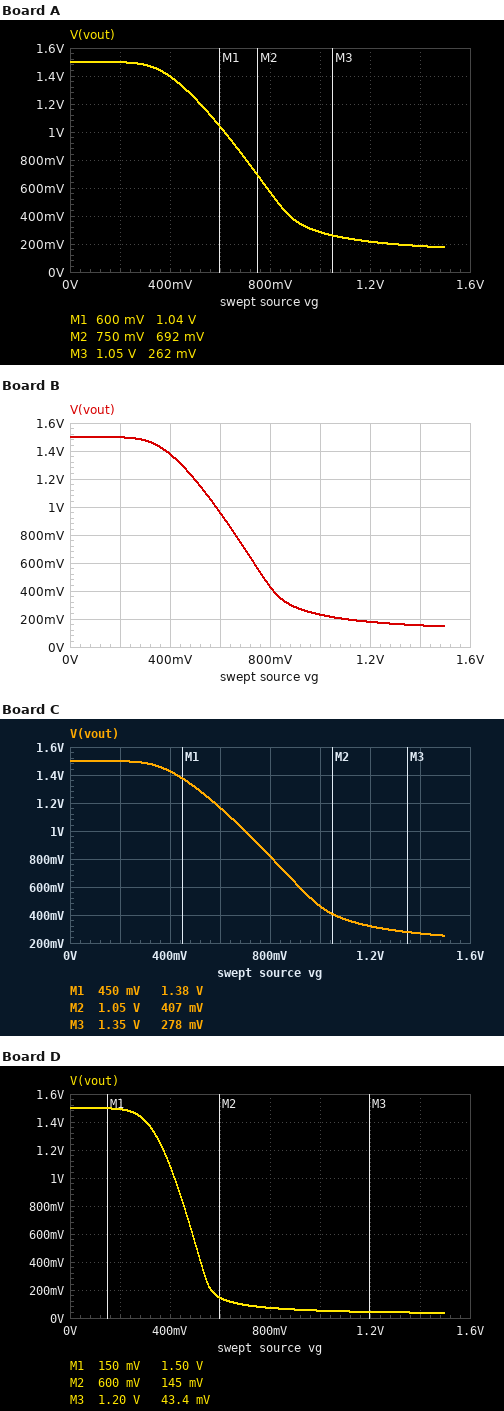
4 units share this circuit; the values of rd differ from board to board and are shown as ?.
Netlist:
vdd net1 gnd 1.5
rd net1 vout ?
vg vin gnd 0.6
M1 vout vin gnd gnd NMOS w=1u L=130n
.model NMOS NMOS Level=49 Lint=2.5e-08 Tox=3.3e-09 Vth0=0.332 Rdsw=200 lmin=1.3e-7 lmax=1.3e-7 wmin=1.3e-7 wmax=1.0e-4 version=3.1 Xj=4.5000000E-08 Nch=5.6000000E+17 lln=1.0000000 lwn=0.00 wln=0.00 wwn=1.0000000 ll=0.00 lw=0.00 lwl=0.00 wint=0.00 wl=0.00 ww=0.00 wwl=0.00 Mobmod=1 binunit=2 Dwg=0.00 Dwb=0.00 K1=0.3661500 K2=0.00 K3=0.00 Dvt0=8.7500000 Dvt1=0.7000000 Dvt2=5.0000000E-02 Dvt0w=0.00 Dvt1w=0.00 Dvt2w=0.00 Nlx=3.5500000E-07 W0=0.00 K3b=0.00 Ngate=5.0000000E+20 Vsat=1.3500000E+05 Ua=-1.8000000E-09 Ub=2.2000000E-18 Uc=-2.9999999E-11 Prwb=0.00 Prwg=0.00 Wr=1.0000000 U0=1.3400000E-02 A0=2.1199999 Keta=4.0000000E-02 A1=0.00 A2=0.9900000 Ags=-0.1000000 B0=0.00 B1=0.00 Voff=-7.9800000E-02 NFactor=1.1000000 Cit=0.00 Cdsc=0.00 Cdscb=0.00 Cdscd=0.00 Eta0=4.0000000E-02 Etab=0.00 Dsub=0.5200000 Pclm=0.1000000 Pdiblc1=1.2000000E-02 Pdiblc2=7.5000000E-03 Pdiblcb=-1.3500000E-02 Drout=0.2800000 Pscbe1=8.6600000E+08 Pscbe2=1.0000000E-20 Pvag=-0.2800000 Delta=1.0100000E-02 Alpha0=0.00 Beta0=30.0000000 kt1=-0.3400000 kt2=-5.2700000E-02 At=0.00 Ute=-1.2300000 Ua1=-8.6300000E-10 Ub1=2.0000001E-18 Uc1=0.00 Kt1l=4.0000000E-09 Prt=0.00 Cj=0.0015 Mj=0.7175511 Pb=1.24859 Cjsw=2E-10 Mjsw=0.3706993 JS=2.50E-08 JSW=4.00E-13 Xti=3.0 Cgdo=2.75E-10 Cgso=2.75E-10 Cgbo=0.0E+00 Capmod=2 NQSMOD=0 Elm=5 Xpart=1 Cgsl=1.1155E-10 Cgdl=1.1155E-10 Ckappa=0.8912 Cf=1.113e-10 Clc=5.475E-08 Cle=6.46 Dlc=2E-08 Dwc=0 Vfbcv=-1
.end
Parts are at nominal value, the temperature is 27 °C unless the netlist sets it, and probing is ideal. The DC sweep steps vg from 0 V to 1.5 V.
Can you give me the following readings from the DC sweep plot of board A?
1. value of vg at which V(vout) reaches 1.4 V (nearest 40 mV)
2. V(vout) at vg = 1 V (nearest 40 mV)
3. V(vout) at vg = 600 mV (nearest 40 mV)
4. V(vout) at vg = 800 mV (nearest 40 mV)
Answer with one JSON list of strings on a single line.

["400 mV", "280 mV", "1.04 V", "560 mV"]
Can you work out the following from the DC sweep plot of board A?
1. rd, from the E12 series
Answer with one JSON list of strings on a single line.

["4.7 kΩ"]
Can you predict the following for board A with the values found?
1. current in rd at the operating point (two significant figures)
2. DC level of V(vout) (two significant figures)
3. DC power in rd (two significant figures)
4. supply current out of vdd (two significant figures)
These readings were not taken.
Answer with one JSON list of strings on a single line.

["98 µA", "1.0 V", "45 µW", "98 µA"]
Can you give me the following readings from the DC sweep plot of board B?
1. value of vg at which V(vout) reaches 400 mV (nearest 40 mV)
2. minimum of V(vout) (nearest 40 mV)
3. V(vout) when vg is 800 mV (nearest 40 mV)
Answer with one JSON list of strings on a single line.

["800 mV", "160 mV", "440 mV"]
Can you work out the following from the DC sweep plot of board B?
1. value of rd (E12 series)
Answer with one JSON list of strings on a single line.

["5.6 kΩ"]
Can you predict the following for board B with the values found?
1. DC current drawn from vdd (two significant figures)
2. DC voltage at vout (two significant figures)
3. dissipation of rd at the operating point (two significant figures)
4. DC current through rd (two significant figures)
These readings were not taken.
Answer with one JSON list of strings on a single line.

["96 µA", "960 mV", "52 µW", "96 µA"]
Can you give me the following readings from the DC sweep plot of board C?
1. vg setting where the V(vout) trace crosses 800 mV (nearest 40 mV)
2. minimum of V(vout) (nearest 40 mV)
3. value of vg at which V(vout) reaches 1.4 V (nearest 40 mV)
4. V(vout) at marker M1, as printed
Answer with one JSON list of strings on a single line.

["800 mV", "240 mV", "440 mV", "1.38 V"]
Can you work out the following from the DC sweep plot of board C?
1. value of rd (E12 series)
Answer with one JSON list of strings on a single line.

["3.3 kΩ"]
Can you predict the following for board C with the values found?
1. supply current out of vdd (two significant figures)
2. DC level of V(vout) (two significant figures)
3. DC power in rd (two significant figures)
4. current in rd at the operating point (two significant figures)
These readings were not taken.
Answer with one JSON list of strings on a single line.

["100 µA", "1.2 V", "34 µW", "100 µA"]
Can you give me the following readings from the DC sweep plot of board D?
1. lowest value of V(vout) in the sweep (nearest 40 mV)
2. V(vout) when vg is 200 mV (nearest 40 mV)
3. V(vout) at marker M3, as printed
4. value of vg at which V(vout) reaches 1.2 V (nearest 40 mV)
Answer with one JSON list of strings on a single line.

["40 mV", "1.48 V", "43.4 mV", "360 mV"]
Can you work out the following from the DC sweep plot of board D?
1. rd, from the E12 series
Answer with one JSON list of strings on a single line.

["22 kΩ"]
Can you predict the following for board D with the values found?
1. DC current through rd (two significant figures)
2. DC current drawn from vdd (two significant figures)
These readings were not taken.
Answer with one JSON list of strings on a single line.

["62 µA", "62 µA"]
